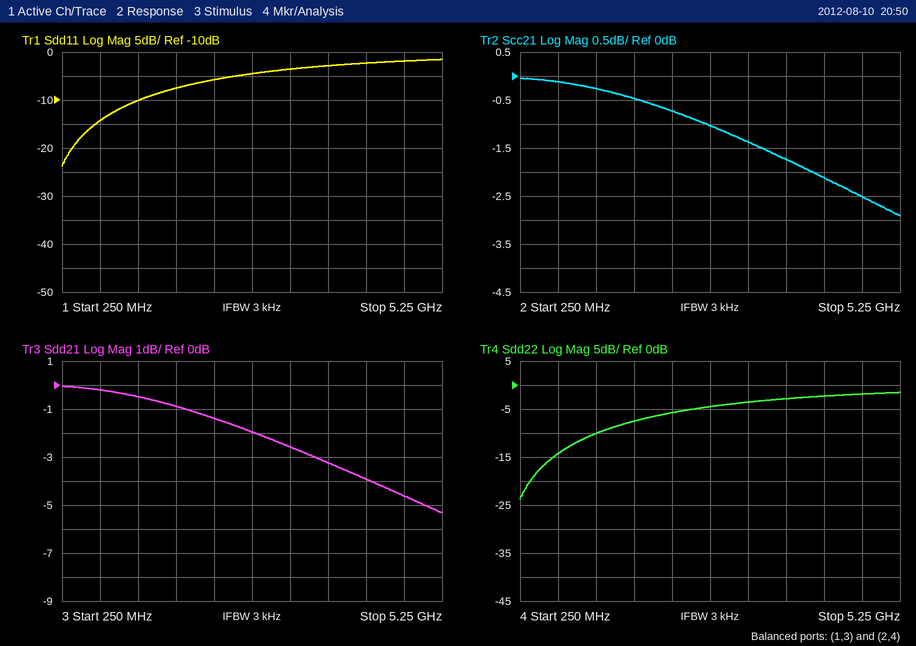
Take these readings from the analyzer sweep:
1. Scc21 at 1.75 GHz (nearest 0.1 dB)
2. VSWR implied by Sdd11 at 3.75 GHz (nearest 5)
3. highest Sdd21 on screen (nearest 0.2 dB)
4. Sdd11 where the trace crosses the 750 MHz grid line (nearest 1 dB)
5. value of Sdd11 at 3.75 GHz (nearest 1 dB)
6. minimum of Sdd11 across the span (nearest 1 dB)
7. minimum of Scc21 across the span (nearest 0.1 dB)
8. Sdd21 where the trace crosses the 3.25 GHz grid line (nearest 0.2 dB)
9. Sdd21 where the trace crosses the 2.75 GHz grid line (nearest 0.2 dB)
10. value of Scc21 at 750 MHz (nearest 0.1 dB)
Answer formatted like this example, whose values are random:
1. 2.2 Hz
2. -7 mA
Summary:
1. -0.5 dB
2. 5
3. 0.0 dB
4. -14 dB
5. -3 dB
6. -24 dB
7. -2.9 dB
8. -2.6 dB
9. -2.0 dB
10. -0.1 dB
